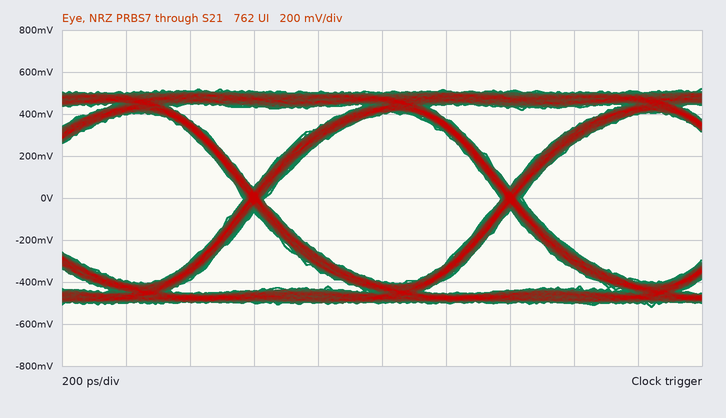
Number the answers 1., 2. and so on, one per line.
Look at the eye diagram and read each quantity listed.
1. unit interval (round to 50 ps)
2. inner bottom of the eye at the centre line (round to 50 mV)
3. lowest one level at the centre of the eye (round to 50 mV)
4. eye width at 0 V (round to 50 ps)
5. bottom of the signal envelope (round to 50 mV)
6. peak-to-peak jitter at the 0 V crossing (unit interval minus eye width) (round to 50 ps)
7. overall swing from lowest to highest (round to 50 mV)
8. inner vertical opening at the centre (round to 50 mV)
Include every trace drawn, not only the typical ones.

1. 800 ps
2. -400 mV
3. 400 mV
4. 750 ps
5. -500 mV
6. 50 ps
7. 1.05 V
8. 800 mV
